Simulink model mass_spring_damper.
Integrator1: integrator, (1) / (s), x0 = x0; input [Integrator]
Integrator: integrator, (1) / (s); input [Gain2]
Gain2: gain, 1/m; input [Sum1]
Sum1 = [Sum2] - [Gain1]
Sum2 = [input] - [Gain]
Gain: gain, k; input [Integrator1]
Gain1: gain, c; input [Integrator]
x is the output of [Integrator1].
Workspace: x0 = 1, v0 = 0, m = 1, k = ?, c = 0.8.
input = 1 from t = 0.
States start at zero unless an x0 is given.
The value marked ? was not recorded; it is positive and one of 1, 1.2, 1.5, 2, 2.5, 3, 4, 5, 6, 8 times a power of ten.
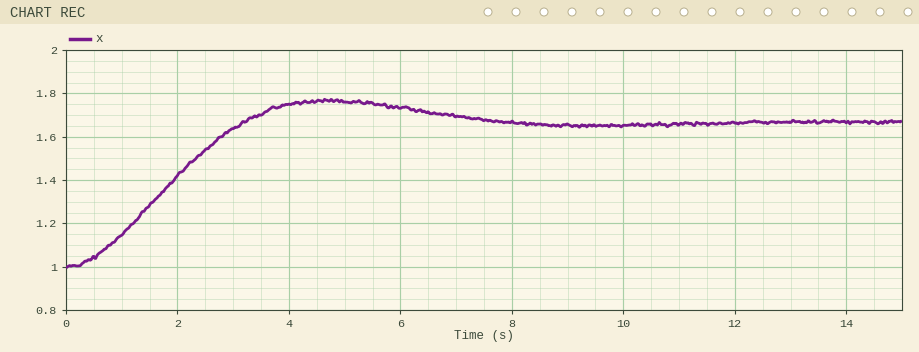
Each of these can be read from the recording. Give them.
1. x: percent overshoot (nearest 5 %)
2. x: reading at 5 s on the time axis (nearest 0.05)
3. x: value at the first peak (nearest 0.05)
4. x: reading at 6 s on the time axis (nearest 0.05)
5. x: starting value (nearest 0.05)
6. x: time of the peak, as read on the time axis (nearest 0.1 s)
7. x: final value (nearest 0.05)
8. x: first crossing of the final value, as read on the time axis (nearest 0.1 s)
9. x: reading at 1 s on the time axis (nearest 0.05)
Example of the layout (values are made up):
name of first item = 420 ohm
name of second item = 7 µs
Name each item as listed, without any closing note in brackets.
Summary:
x: percent overshoot = 15 %
x: reading at 5 s on the time axis = 1.75
x: value at the first peak = 1.75
x: reading at 6 s on the time axis = 1.75
x: starting value = 1.00
x: time of the peak, as read on the time axis = 4.7 s
x: final value = 1.65
x: first crossing of the final value, as read on the time axis = 3.2 s
x: reading at 1 s on the time axis = 1.15
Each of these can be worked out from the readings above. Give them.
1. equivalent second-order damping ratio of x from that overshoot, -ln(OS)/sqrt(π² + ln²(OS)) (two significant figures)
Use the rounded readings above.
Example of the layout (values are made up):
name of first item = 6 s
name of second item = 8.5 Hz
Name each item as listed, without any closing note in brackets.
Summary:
equivalent second-order damping ratio of x from that overshoot, -ln(OS)/sqrt(π² + ln²(OS)) = 0.52
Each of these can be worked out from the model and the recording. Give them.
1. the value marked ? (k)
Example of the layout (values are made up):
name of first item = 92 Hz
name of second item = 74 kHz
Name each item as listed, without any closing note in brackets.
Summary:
the value marked ? = 0.6
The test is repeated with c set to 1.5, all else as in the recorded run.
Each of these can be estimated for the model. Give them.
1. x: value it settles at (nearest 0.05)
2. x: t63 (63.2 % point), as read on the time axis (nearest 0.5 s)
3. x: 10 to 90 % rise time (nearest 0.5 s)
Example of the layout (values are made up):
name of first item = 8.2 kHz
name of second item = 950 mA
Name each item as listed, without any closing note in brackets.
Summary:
x: value it settles at = 1.65
x: t63 (63.2 % point), as read on the time axis = 2.5 s
x: 10 to 90 % rise time = 4.0 s
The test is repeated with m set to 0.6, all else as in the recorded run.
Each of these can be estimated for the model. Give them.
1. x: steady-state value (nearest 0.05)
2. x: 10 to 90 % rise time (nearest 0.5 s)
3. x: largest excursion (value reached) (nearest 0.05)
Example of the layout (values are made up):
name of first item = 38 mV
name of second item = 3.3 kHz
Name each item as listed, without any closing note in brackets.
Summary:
x: steady-state value = 1.65
x: 10 to 90 % rise time = 2.0 s
x: largest excursion (value reached) = 1.70
